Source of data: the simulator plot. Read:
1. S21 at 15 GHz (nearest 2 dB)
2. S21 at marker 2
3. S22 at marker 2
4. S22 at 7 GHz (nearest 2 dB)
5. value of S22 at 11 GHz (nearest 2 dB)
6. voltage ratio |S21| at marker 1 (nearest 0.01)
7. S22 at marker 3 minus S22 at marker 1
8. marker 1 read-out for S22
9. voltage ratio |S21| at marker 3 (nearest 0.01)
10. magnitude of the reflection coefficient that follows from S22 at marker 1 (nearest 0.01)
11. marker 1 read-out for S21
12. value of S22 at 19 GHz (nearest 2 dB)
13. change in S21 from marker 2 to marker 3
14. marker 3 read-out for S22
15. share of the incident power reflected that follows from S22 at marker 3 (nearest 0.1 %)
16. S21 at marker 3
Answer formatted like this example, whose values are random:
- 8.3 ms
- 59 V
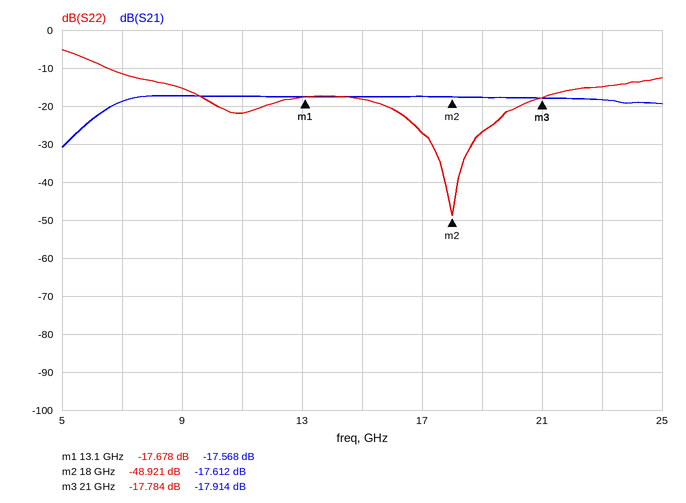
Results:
- -18 dB
- -17.612 dB
- -48.921 dB
- -12 dB
- -22 dB
- 0.13
- -0.106 dB
- -17.678 dB
- 0.13
- 0.13
- -17.568 dB
- -26 dB
- -0.302 dB
- -17.784 dB
- 1.7 %
- -17.914 dB
